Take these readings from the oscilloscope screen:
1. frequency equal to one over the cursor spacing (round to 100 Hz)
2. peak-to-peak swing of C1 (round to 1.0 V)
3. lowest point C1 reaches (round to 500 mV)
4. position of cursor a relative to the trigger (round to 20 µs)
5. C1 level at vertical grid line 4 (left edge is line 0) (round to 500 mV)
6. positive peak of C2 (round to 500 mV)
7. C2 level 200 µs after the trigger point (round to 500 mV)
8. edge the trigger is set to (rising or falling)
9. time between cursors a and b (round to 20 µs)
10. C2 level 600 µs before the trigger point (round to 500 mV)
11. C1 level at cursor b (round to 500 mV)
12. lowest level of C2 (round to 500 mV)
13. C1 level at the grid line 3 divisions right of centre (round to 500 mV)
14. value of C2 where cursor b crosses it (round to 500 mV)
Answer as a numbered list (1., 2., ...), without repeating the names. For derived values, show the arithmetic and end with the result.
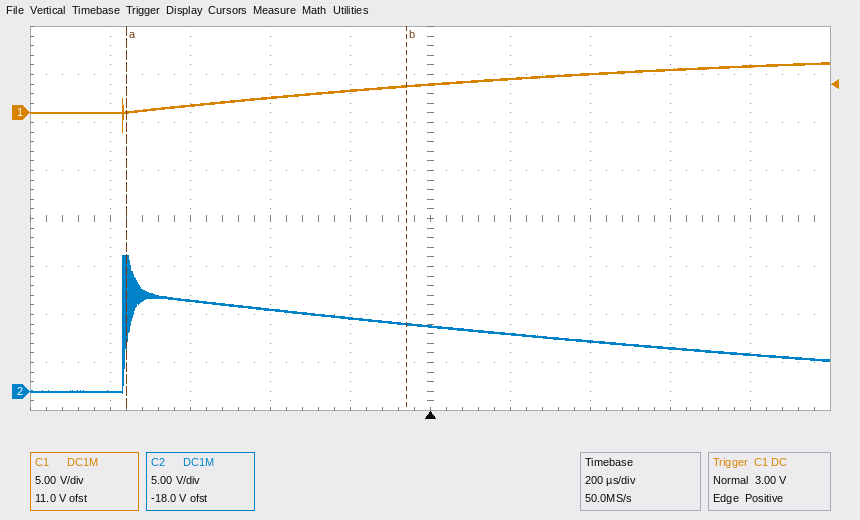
1. 1 / 700 µs ≈ 1.4 kHz
2. 7.0 V
3. -2.0 V
4. -760 µs
5. 2.5 V
6. 14.0 V
7. 6.0 V
8. rising
9. 700 µs
10. 9.5 V
11. 3.0 V
12. 0.0 V
13. 4.5 V
14. 7.0 V
